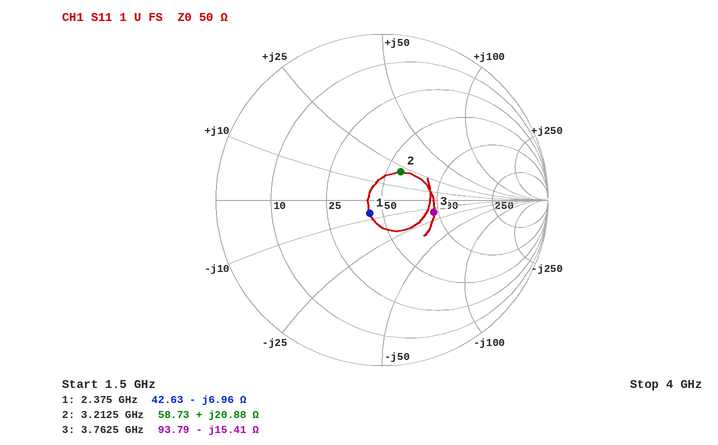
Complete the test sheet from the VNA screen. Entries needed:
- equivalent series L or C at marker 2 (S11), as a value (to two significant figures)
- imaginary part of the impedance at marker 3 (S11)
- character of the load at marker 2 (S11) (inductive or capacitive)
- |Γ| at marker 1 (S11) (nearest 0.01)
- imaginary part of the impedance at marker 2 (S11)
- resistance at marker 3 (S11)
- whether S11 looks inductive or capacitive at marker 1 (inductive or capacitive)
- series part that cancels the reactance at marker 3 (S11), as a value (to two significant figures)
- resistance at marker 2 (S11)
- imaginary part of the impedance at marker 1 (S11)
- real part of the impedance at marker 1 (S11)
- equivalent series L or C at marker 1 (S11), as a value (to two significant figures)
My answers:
1.0 nH
-15.41 Ω
inductive
0.11
+20.88 Ω
93.79 Ω
capacitive
650 pH
58.73 Ω
-6.96 Ω
42.63 Ω
9.6 pF
